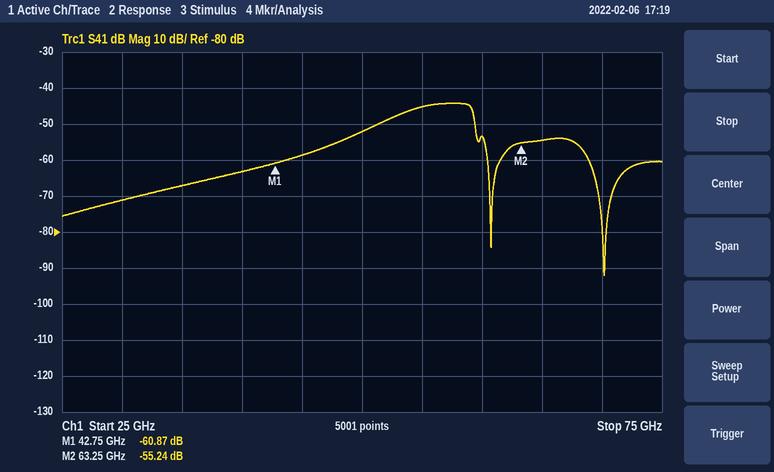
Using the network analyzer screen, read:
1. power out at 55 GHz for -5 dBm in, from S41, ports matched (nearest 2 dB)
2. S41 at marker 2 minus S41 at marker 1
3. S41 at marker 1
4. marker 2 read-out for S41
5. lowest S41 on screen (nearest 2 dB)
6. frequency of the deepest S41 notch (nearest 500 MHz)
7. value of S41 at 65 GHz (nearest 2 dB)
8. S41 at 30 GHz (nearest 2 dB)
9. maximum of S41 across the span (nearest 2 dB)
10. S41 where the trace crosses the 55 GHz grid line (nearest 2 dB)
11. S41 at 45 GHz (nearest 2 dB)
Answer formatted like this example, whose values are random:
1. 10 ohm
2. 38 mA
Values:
1. -50 dBm
2. 5.63 dB
3. -60.87 dB
4. -55.24 dB
5. -92 dB
6. 70.0 GHz
7. -54 dB
8. -72 dB
9. -44 dB
10. -46 dB
11. -58 dB
